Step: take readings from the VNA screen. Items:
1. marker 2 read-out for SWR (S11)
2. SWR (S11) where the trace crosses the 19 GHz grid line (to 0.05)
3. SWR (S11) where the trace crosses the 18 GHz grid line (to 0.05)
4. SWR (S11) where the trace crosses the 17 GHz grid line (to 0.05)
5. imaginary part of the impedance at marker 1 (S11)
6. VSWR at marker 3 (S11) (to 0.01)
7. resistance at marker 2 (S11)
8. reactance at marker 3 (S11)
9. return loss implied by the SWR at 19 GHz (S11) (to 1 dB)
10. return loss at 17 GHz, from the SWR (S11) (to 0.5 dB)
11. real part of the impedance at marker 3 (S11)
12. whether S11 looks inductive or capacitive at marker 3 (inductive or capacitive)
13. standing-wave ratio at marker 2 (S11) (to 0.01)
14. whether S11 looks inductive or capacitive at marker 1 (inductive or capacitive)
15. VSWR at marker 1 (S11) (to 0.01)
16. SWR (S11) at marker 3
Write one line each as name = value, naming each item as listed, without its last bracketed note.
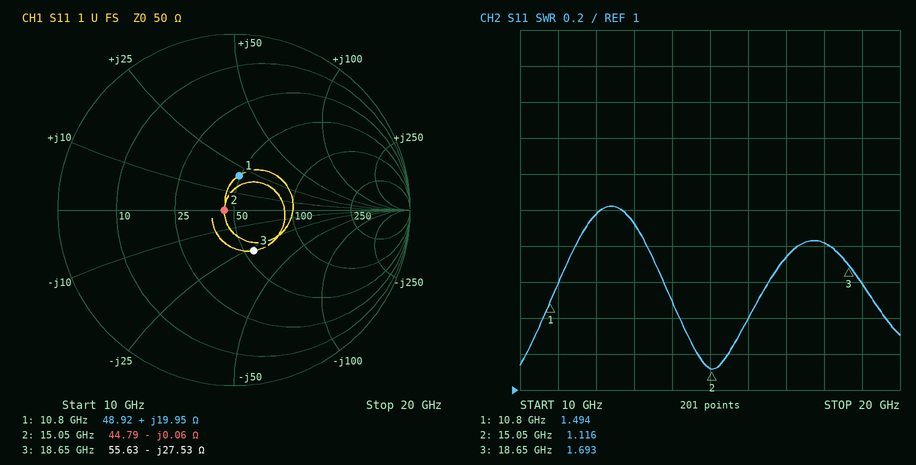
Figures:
marker 2 read-out for SWR = 1.116
SWR (S11) where the trace crosses the 19 GHz grid line = 1.60
SWR (S11) where the trace crosses the 18 GHz grid line = 1.80
SWR (S11) where the trace crosses the 17 GHz grid line = 1.75
imaginary part of the impedance at marker 1 = +19.95 Ω
VSWR at marker 3 (S11) = 1.69
resistance at marker 2 = 44.79 Ω
reactance at marker 3 = -27.53 Ω
return loss implied by the SWR at 19 GHz (S11) = 13 dB
return loss at 17 GHz, from the SWR (S11) = 11.5 dB
real part of the impedance at marker 3 = 55.63 Ω
whether S11 looks inductive or capacitive at marker 3 = capacitive
standing-wave ratio at marker 2 (S11) = 1.12
whether S11 looks inductive or capacitive at marker 1 = inductive
VSWR at marker 1 (S11) = 1.49
SWR (S11) at marker 3 = 1.693
